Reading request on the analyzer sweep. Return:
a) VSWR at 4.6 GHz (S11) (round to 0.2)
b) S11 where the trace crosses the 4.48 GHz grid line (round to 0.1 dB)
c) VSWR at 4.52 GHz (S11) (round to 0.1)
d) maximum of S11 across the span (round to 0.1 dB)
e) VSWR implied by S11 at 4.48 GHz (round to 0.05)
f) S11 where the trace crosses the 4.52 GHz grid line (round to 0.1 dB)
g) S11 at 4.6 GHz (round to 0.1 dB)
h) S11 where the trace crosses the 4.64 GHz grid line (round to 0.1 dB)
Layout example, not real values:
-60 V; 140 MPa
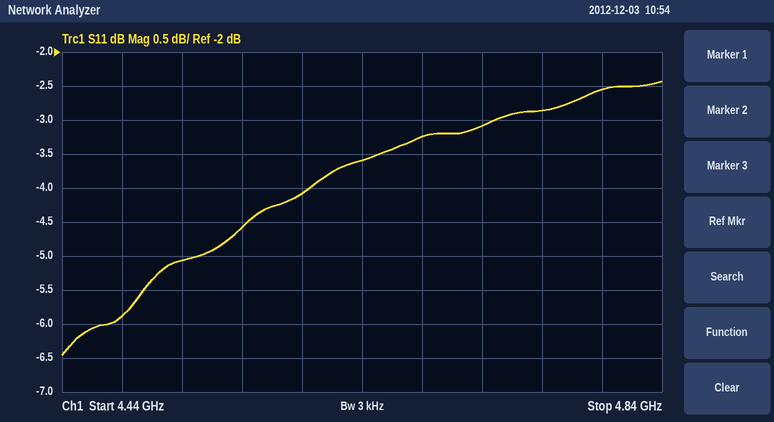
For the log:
4.4; -5.9 dB; 3.5; -2.4 dB; 3.05; -5.1 dB; -4.1 dB; -3.6 dB
